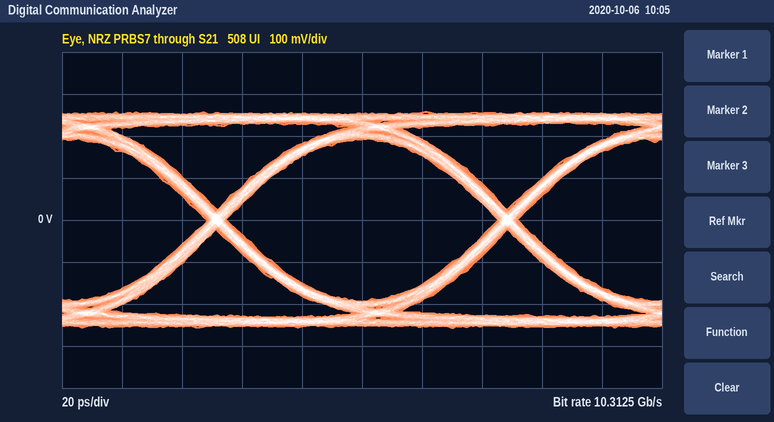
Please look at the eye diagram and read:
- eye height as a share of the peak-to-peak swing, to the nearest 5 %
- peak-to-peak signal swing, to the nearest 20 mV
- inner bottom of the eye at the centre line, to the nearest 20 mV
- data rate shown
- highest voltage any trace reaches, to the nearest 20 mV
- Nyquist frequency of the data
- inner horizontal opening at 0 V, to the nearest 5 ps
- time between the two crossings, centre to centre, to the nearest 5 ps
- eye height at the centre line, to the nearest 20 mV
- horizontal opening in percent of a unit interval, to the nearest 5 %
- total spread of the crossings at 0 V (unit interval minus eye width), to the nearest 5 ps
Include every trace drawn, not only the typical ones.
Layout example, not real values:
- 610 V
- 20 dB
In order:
- 75 %
- 520 mV
- -200 mV
- 10.3125 Gb/s
- 260 mV
- 5.15625 GHz
- 90 ps
- 95 ps
- 380 mV
- 95 %
- 5 ps
